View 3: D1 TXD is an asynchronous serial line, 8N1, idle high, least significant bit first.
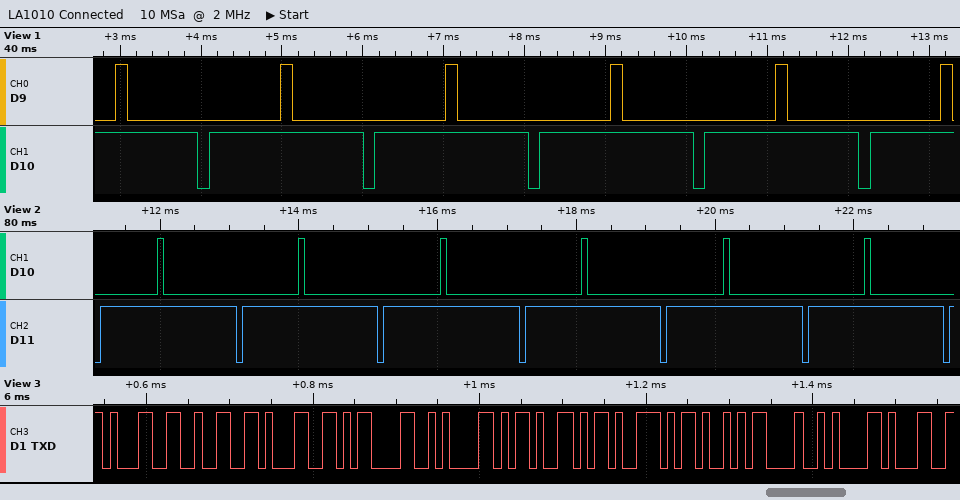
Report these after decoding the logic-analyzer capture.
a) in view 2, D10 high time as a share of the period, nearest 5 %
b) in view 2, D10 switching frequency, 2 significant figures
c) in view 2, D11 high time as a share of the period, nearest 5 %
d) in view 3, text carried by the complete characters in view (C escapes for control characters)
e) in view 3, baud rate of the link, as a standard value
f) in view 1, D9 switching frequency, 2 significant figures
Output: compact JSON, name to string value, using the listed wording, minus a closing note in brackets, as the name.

{"in view 2, D10 high time as a share of the period, nearest 5 %": "5 %", "in view 2, D10 switching frequency, 2 significant figures": "490 Hz", "in view 2, D11 high time as a share of the period, nearest 5 %": "95 %", "in view 3, text carried by the complete characters in view": "\"121\\r\\n---\\r\\n1\"", "in view 3, baud rate of the link, as a standard value": "115200 baud", "in view 1, D9 switching frequency, 2 significant figures": "490 Hz"}
